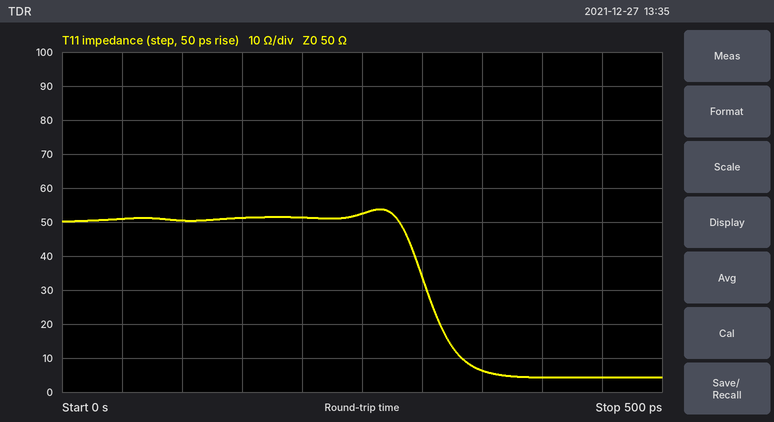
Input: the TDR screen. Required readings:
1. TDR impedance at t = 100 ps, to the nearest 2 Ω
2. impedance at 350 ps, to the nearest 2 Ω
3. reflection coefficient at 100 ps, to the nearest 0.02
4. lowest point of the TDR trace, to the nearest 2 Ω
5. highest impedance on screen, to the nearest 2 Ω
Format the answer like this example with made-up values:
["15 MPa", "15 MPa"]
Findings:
["50 Ω", "6 Ω", "0.00", "4 Ω", "54 Ω"]
